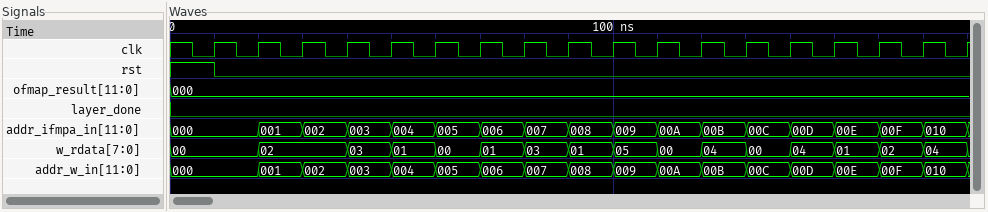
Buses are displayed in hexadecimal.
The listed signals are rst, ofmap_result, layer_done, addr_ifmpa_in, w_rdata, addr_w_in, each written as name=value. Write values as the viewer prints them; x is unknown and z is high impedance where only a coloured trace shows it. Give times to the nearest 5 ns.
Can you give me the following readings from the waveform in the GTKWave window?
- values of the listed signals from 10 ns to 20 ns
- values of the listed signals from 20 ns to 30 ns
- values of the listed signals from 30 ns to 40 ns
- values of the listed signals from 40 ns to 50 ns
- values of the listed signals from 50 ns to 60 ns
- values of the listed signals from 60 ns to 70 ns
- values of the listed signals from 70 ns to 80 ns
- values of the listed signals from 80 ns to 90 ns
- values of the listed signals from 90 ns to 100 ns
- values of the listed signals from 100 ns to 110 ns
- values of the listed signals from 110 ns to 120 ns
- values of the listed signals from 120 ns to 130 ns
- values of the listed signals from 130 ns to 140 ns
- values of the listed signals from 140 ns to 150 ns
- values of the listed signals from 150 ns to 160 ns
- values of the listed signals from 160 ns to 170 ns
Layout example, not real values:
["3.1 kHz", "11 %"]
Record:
["rst=0, ofmap_result=000, layer_done=0, addr_ifmpa_in=000, w_rdata=00, addr_w_in=000", "rst=0, ofmap_result=000, layer_done=0, addr_ifmpa_in=001, w_rdata=02, addr_w_in=001", "rst=0, ofmap_result=000, layer_done=0, addr_ifmpa_in=002, w_rdata=02, addr_w_in=002", "rst=0, ofmap_result=000, layer_done=0, addr_ifmpa_in=003, w_rdata=03, addr_w_in=003", "rst=0, ofmap_result=000, layer_done=0, addr_ifmpa_in=004, w_rdata=01, addr_w_in=004", "rst=0, ofmap_result=000, layer_done=0, addr_ifmpa_in=005, w_rdata=00, addr_w_in=005", "rst=0, ofmap_result=000, layer_done=0, addr_ifmpa_in=006, w_rdata=01, addr_w_in=006", "rst=0, ofmap_result=000, layer_done=0, addr_ifmpa_in=007, w_rdata=03, addr_w_in=007", "rst=0, ofmap_result=000, layer_done=0, addr_ifmpa_in=008, w_rdata=01, addr_w_in=008", "rst=0, ofmap_result=000, layer_done=0, addr_ifmpa_in=009, w_rdata=05, addr_w_in=009", "rst=0, ofmap_result=000, layer_done=0, addr_ifmpa_in=00A, w_rdata=00, addr_w_in=00A", "rst=0, ofmap_result=000, layer_done=0, addr_ifmpa_in=00B, w_rdata=04, addr_w_in=00B", "rst=0, ofmap_result=000, layer_done=0, addr_ifmpa_in=00C, w_rdata=00, addr_w_in=00C", "rst=0, ofmap_result=000, layer_done=0, addr_ifmpa_in=00D, w_rdata=04, addr_w_in=00D", "rst=0, ofmap_result=000, layer_done=0, addr_ifmpa_in=00E, w_rdata=01, addr_w_in=00E", "rst=0, ofmap_result=000, layer_done=0, addr_ifmpa_in=00F, w_rdata=02, addr_w_in=00F"]
